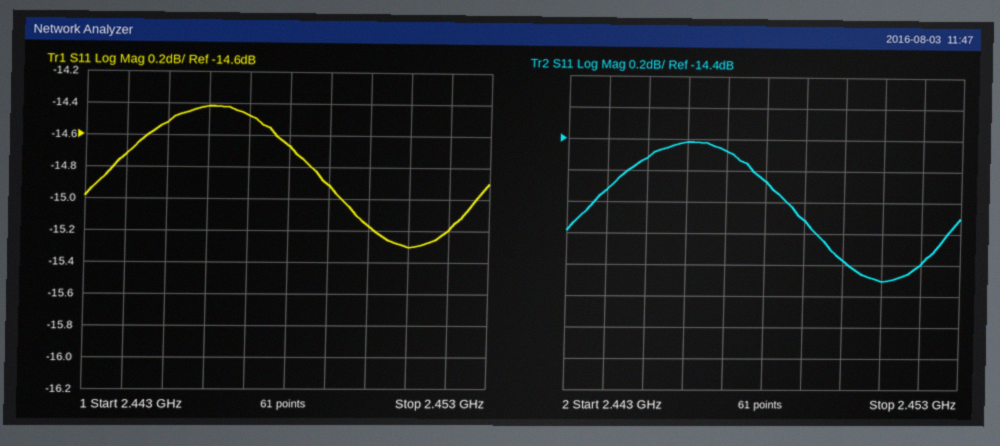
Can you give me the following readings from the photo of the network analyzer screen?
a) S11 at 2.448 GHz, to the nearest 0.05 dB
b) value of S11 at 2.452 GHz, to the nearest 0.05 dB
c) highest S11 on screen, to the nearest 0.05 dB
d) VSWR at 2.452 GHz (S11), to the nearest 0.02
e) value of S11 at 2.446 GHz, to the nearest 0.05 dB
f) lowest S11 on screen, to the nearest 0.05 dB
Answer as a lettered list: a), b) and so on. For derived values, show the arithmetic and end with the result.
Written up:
a) -14.65 dB
b) -15.20 dB
c) -14.40 dB
d) |Γ| = 10^(-15.2/20) = 0.1738; VSWR = (1 + 0.1738)/(1 − 0.1738) ≈ 1.42
e) -14.40 dB
f) -15.30 dB
